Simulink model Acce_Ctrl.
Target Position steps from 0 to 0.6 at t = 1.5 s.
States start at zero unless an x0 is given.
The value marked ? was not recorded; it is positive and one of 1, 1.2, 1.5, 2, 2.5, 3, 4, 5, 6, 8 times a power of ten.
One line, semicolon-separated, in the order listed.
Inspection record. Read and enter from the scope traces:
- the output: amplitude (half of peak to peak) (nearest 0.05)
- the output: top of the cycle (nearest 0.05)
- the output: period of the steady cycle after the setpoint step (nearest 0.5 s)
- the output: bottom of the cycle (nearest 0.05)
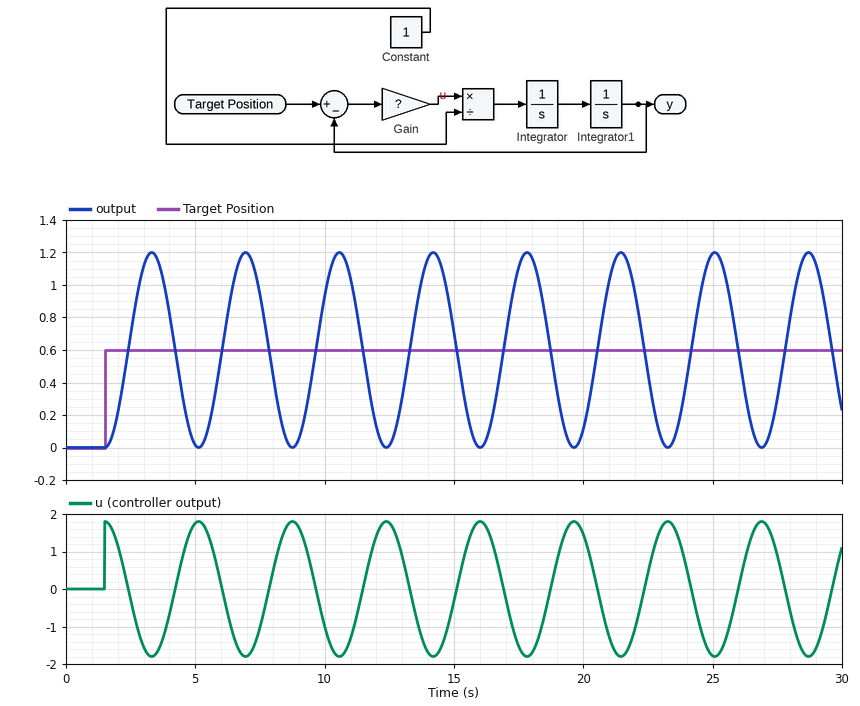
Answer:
0.60; 1.20; 3.5 s; 0.00
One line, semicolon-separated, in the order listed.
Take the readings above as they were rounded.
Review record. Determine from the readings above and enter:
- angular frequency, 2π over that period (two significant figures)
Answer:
1.8 rad/s
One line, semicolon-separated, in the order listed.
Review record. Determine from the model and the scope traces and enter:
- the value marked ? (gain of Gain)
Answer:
3
